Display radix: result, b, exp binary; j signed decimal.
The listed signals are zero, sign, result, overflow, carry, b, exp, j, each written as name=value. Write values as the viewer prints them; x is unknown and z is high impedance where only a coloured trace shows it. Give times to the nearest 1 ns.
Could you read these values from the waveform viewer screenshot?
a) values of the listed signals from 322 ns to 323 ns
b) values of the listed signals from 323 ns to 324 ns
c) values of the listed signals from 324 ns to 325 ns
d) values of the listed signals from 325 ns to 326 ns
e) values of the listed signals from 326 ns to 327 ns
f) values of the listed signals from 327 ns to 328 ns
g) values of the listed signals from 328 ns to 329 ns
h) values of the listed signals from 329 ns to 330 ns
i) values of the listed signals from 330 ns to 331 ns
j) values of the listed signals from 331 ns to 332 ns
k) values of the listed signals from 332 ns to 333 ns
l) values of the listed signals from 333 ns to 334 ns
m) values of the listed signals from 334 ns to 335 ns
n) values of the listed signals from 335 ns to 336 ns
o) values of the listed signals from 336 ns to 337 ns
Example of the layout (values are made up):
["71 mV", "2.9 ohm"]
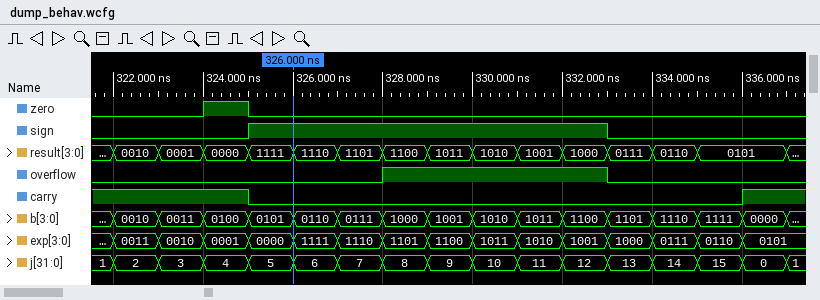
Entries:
["zero=0, sign=0, result=0010, overflow=0, carry=1, b=0010, exp=0011, j=2", "zero=0, sign=0, result=0001, overflow=0, carry=1, b=0011, exp=0010, j=3", "zero=1, sign=0, result=0000, overflow=0, carry=1, b=0100, exp=0001, j=4", "zero=0, sign=1, result=1111, overflow=0, carry=0, b=0101, exp=0000, j=5", "zero=0, sign=1, result=1110, overflow=0, carry=0, b=0110, exp=1111, j=6", "zero=0, sign=1, result=1101, overflow=0, carry=0, b=0111, exp=1110, j=7", "zero=0, sign=1, result=1100, overflow=1, carry=0, b=1000, exp=1101, j=8", "zero=0, sign=1, result=1011, overflow=1, carry=0, b=1001, exp=1100, j=9", "zero=0, sign=1, result=1010, overflow=1, carry=0, b=1010, exp=1011, j=10", "zero=0, sign=1, result=1001, overflow=1, carry=0, b=1011, exp=1010, j=11", "zero=0, sign=1, result=1000, overflow=1, carry=0, b=1100, exp=1001, j=12", "zero=0, sign=0, result=0111, overflow=0, carry=0, b=1101, exp=1000, j=13", "zero=0, sign=0, result=0110, overflow=0, carry=0, b=1110, exp=0111, j=14", "zero=0, sign=0, result=0101, overflow=0, carry=0, b=1111, exp=0110, j=15", "zero=0, sign=0, result=0101, overflow=0, carry=1, b=0000, exp=0101, j=0"]
